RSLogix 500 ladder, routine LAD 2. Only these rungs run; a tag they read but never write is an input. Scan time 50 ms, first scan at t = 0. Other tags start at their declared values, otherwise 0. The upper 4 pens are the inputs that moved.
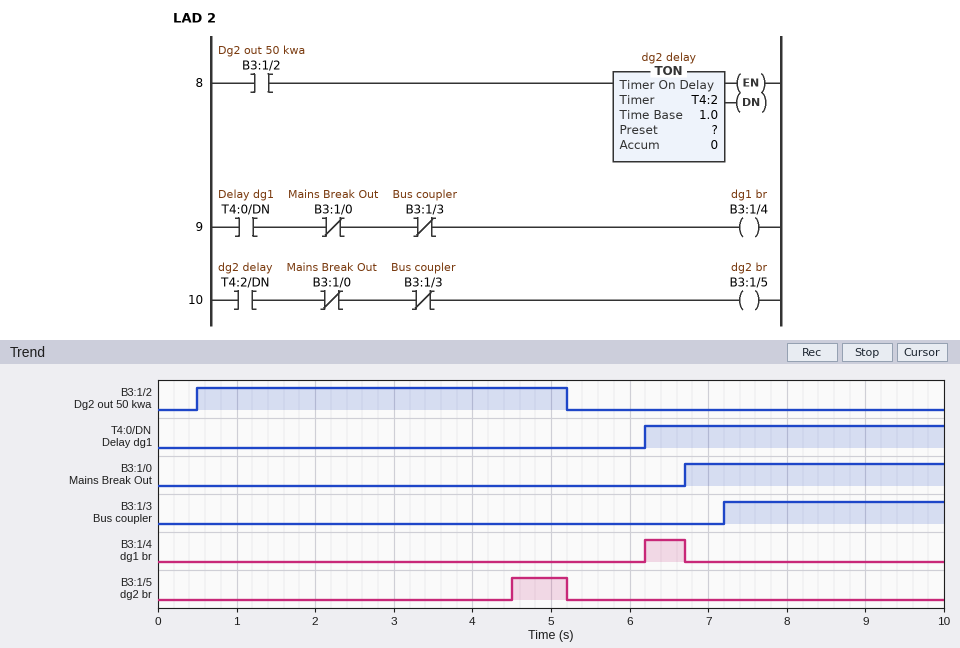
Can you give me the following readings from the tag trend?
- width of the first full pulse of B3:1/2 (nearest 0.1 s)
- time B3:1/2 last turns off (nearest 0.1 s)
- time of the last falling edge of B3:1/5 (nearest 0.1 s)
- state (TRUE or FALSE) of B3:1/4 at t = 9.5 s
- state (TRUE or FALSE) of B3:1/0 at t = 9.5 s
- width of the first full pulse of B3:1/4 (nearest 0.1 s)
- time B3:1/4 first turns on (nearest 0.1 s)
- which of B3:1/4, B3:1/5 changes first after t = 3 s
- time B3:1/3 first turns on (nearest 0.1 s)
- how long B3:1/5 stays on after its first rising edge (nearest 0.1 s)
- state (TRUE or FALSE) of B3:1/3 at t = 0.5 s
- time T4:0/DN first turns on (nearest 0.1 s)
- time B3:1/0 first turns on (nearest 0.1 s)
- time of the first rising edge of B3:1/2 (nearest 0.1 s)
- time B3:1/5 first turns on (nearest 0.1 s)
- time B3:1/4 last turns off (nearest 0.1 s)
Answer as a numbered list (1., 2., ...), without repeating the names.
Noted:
1. 4.7 s
2. 5.2 s
3. 5.2 s
4. FALSE
5. TRUE
6. 0.5 s
7. 6.2 s
8. B3:1/5
9. 7.2 s
10. 0.7 s
11. FALSE
12. 6.2 s
13. 6.7 s
14. 0.5 s
15. 4.5 s
16. 6.7 s
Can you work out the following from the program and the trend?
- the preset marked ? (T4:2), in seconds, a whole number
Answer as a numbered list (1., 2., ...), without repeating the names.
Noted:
1. 4 s
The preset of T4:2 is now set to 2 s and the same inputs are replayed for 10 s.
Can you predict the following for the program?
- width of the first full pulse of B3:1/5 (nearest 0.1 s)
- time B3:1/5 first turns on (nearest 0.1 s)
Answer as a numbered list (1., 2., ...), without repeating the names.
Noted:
1. 2.7 s
2. 2.5 s
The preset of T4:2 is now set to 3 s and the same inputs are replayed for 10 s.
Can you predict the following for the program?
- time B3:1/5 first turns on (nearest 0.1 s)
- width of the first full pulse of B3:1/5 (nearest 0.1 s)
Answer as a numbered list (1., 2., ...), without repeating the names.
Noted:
1. 3.5 s
2. 1.7 s
